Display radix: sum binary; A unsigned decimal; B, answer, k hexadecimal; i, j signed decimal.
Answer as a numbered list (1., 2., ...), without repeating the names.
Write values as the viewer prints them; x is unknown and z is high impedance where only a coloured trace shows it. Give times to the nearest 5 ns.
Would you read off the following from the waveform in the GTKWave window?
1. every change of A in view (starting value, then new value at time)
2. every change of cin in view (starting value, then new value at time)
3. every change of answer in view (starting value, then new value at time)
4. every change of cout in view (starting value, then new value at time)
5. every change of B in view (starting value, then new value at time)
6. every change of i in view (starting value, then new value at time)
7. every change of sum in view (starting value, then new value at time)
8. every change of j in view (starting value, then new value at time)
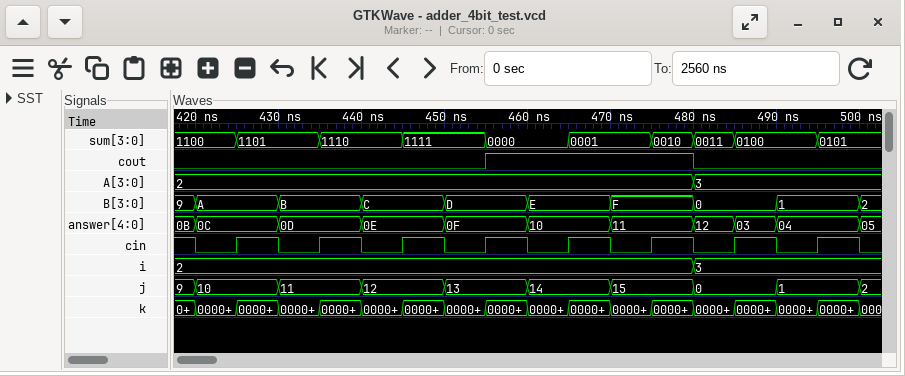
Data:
1. 2, 3 at 480 ns
2. 1, 0 at 420 ns, 1 at 425 ns, 0 at 430 ns, 1 at 435 ns, 0 at 440 ns, 1 at 445 ns, 0 at 450 ns, 1 at 455 ns, 0 at 460 ns, 1 at 465 ns, 0 at 470 ns, 1 at 475 ns, 0 at 480 ns, 1 at 485 ns, 0 at 490 ns, 1 at 495 ns, 0 at 500 ns
3. 0B, 0C at 420 ns, 0D at 430 ns, 0E at 440 ns, 0F at 450 ns, 10 at 460 ns, 11 at 470 ns, 12 at 480 ns, 03 at 485 ns, 04 at 490 ns, 05 at 500 ns
4. 0, 1 at 455 ns, 0 at 480 ns
5. 9, A at 420 ns, B at 430 ns, C at 440 ns, D at 450 ns, E at 460 ns, F at 470 ns, 0 at 480 ns, 1 at 490 ns, 2 at 500 ns
6. 2, 3 at 480 ns
7. 1100, 1101 at 425 ns, 1110 at 435 ns, 1111 at 445 ns, 0000 at 455 ns, 0001 at 465 ns, 0010 at 475 ns, 0011 at 480 ns, 0100 at 485 ns, 0101 at 495 ns
8. 9, 10 at 420 ns, 11 at 430 ns, 12 at 440 ns, 13 at 450 ns, 14 at 460 ns, 15 at 470 ns, 0 at 480 ns, 1 at 490 ns, 2 at 500 ns
